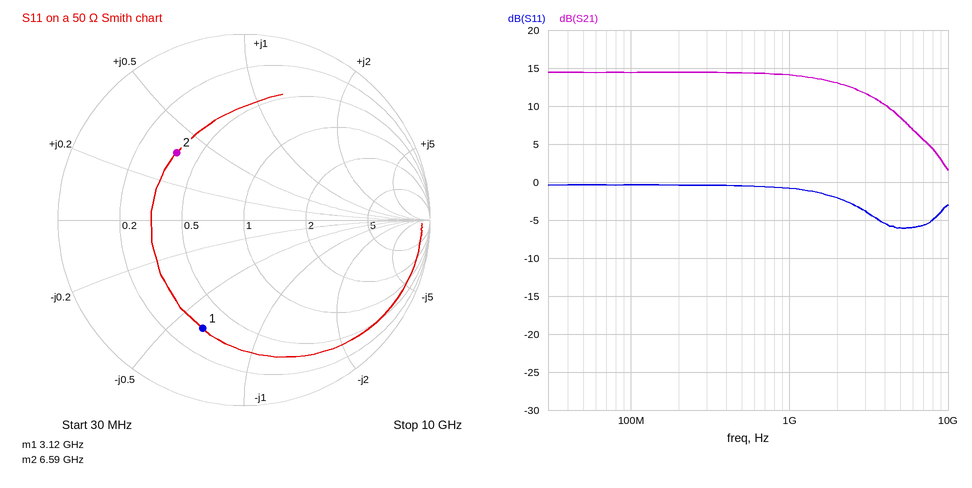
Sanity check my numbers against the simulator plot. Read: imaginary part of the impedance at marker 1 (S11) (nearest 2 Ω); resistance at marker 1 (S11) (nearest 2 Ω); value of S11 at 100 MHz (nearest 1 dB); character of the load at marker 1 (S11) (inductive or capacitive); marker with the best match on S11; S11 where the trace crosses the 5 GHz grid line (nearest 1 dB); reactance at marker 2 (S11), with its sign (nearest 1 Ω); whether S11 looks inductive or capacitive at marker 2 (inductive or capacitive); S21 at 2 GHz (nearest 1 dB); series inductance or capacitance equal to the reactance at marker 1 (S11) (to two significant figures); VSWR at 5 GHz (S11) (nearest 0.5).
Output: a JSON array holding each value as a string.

["-32 Ω", "16 Ω", "0 dB", "capacitive", "marker 2", "-6 dB", "+18 Ω", "inductive", "13 dB", "1.6 pF", "3.0"]
